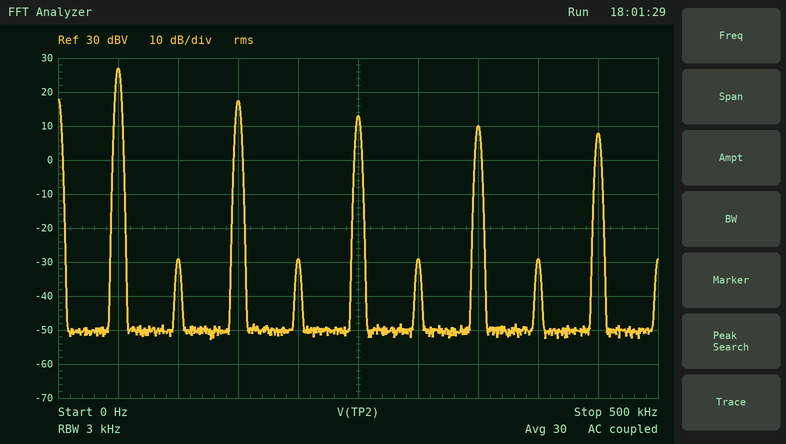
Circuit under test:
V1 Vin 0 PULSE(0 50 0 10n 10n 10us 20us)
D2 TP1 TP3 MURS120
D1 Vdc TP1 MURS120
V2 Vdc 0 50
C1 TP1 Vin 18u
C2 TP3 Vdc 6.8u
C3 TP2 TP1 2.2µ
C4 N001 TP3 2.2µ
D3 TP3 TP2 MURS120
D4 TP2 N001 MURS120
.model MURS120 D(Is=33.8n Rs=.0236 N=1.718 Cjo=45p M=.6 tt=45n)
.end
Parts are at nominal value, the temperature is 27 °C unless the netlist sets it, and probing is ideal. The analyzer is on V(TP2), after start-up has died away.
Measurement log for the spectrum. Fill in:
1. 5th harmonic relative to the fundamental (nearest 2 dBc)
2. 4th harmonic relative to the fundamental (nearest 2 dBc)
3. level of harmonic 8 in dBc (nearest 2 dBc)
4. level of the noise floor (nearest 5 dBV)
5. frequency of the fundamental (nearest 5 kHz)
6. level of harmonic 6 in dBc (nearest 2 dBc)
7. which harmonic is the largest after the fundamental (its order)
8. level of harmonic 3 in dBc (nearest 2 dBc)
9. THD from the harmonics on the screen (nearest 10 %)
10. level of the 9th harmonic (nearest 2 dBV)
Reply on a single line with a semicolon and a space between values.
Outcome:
-14 dBc; -56 dBc; -56 dBc; -50 dBV; 50 kHz; -56 dBc; 3; -10 dBc; 40 %; 8 dBV
